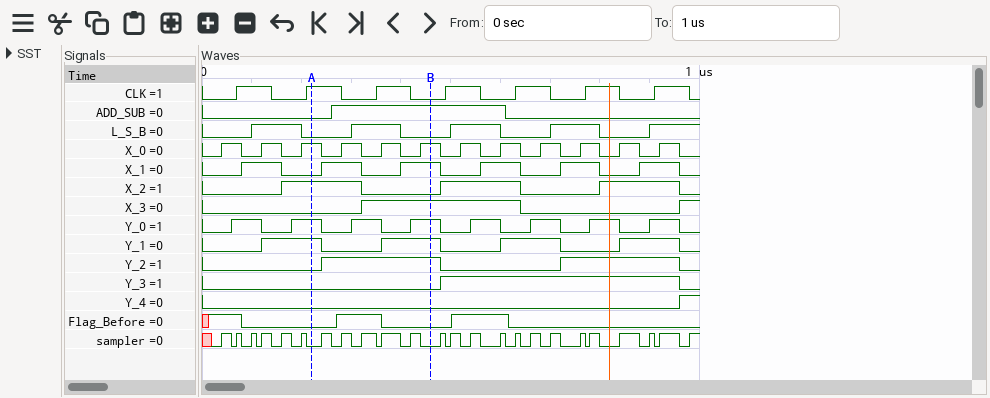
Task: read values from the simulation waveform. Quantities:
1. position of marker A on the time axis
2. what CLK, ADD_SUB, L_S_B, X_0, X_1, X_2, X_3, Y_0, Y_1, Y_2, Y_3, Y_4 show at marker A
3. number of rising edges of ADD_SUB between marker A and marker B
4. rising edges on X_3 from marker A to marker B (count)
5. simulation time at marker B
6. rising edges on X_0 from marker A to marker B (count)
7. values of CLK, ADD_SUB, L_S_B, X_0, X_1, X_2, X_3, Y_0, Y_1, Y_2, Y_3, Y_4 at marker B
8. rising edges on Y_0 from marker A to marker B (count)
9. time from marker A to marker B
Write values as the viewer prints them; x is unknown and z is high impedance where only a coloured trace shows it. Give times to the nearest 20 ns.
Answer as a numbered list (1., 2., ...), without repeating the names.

1. 220 ns
2. CLK=1, ADD_SUB=0, L_S_B=0, X_0=1, X_1=0, X_2=1, X_3=0, Y_0=1, Y_1=1, Y_2=0, Y_3=0, Y_4=0
3. 1
4. 1
5. 460 ns
6. 3
7. CLK=0, ADD_SUB=1, L_S_B=0, X_0=1, X_1=1, X_2=0, X_3=1, Y_0=1, Y_1=1, Y_2=1, Y_3=0, Y_4=0
8. 2
9. 240 ns
